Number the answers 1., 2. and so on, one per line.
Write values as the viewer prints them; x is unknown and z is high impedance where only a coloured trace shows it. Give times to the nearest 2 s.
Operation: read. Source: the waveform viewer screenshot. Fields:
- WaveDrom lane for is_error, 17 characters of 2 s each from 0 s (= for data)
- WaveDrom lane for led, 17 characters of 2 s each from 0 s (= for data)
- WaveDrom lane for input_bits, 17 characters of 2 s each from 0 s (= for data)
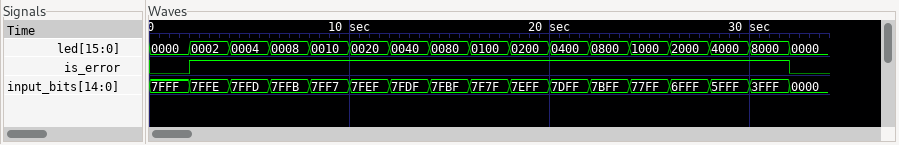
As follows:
1. {name: 'is_error', wave: '01..............0'}
2. {name: 'led', wave: '=================', data: '0000 0002 0004 0008 0010 0020 0040 0080 0100 0200 0400 0800 1000 2000 4000 8000 0000'}
3. {name: 'input_bits', wave: '=================', data: '7FFF 7FFE 7FFD 7FFB 7FF7 7FEF 7FDF 7FBF 7F7F 7EFF 7DFF 7BFF 77FF 6FFF 5FFF 3FFF 0000'}
